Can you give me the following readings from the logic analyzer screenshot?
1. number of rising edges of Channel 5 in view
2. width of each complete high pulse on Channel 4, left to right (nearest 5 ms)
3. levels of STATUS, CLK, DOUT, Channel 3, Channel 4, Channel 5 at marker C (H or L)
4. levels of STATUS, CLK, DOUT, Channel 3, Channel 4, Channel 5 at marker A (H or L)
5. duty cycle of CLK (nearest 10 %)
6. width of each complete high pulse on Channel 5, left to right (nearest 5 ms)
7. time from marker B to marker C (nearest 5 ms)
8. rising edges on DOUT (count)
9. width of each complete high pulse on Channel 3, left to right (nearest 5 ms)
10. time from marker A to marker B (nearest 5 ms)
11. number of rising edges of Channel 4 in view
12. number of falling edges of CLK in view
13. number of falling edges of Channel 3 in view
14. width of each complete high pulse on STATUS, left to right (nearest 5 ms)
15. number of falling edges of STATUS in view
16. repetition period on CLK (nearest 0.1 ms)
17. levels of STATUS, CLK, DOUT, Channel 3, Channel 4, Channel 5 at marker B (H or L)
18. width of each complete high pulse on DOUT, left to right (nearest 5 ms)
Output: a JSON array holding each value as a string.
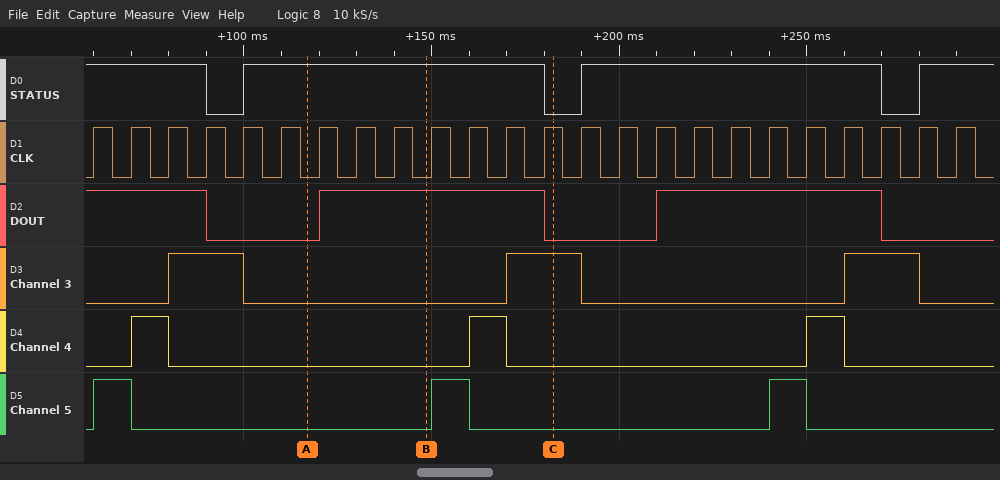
["3", "10 ms, 10 ms, 10 ms", "STATUS=L, CLK=H, DOUT=L, Channel 3=H, Channel 4=L, Channel 5=L", "STATUS=H, CLK=L, DOUT=L, Channel 3=L, Channel 4=L, Channel 5=L", "50 %", "10 ms, 10 ms, 10 ms", "35 ms", "2", "20 ms, 20 ms, 20 ms", "30 ms", "3", "24", "3", "80 ms, 80 ms", "3", "10 ms", "STATUS=H, CLK=L, DOUT=H, Channel 3=L, Channel 4=L, Channel 5=L", "60 ms, 60 ms"]
